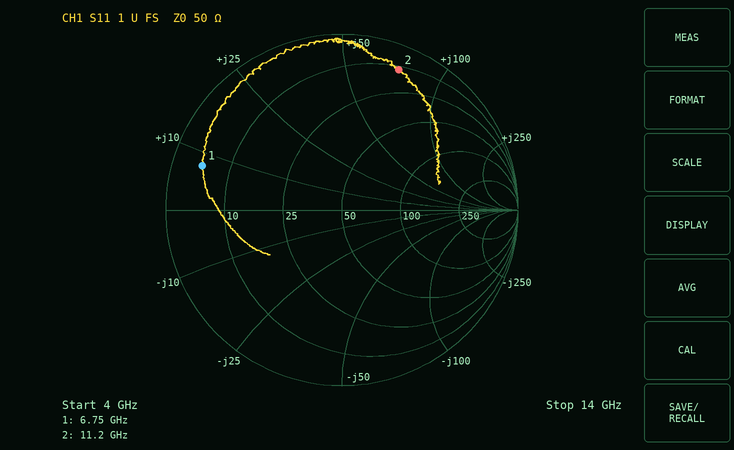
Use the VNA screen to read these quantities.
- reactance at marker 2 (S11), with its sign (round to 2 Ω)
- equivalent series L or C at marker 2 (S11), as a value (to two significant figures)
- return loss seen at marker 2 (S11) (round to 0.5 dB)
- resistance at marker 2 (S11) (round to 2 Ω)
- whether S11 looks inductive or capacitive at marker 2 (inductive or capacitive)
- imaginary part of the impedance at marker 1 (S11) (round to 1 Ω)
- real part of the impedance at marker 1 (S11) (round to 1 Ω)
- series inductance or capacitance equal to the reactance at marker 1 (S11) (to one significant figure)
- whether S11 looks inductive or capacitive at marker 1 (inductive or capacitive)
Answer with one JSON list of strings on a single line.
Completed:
["+72 Ω", "1.0 nH", "1.5 dB", "12 Ω", "inductive", "+8 Ω", "5 Ω", "200 pH", "inductive"]
